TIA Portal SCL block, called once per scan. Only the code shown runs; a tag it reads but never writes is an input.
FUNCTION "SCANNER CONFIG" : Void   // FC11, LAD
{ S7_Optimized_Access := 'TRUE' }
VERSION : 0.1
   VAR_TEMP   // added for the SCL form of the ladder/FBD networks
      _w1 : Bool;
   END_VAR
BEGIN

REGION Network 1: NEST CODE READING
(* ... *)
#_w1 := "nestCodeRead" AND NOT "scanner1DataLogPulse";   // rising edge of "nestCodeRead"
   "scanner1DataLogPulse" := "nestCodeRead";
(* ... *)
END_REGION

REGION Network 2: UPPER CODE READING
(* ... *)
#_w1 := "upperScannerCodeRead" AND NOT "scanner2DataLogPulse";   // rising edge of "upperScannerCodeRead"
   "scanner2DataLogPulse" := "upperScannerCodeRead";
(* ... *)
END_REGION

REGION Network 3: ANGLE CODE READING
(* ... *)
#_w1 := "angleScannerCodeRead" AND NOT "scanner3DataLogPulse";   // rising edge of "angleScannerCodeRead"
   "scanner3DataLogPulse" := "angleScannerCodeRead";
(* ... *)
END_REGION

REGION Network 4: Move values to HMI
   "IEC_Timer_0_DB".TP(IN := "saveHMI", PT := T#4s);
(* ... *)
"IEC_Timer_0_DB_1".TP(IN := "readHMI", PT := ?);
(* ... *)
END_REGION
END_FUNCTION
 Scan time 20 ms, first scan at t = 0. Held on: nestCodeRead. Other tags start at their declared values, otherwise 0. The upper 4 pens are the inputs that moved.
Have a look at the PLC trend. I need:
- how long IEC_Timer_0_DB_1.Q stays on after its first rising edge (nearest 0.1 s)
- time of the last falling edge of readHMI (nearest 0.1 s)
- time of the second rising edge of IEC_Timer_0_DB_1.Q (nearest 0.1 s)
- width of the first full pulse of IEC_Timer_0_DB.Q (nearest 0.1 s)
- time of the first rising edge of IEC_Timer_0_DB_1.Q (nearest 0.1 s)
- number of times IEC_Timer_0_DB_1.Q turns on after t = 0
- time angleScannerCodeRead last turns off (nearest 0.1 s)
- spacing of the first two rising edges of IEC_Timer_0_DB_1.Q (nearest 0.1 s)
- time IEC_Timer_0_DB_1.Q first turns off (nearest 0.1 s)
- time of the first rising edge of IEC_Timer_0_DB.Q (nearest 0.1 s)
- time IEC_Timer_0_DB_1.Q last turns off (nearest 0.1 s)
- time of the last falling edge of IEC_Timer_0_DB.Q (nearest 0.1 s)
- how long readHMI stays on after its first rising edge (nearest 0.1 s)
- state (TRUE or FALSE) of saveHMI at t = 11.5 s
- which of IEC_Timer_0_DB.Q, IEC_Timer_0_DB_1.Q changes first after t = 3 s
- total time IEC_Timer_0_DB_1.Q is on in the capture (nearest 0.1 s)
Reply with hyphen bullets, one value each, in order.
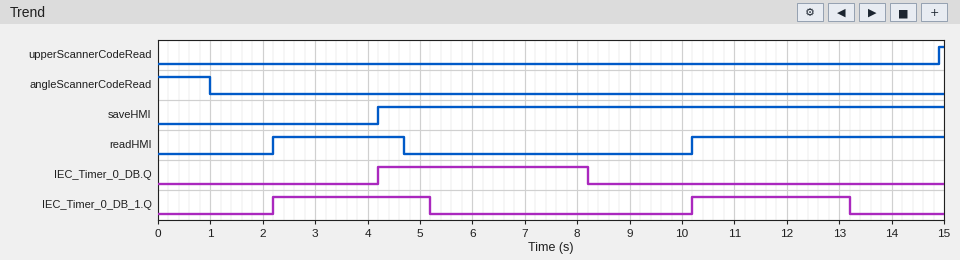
- 3.0 s
- 4.7 s
- 10.2 s
- 4.0 s
- 2.2 s
- 2
- 1.0 s
- 8.0 s
- 5.2 s
- 4.2 s
- 13.2 s
- 8.2 s
- 2.5 s
- TRUE
- IEC_Timer_0_DB.Q
- 6.0 s
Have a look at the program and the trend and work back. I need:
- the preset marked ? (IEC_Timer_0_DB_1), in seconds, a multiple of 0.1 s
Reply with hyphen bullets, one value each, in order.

- 3.0 s
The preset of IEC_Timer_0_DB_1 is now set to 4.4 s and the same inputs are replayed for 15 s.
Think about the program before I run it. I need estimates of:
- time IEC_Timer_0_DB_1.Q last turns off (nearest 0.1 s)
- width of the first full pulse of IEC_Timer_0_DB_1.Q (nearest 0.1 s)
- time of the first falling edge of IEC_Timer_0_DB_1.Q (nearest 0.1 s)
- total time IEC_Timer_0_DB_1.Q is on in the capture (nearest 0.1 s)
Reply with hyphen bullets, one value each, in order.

- 14.6 s
- 4.4 s
- 6.6 s
- 8.8 s
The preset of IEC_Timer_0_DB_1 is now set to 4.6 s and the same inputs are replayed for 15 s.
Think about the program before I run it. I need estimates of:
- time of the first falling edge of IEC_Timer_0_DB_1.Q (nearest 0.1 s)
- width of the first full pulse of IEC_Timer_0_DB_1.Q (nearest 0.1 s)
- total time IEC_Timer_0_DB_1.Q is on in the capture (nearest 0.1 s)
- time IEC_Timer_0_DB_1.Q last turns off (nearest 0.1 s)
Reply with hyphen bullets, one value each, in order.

- 6.8 s
- 4.6 s
- 9.2 s
- 14.8 s
